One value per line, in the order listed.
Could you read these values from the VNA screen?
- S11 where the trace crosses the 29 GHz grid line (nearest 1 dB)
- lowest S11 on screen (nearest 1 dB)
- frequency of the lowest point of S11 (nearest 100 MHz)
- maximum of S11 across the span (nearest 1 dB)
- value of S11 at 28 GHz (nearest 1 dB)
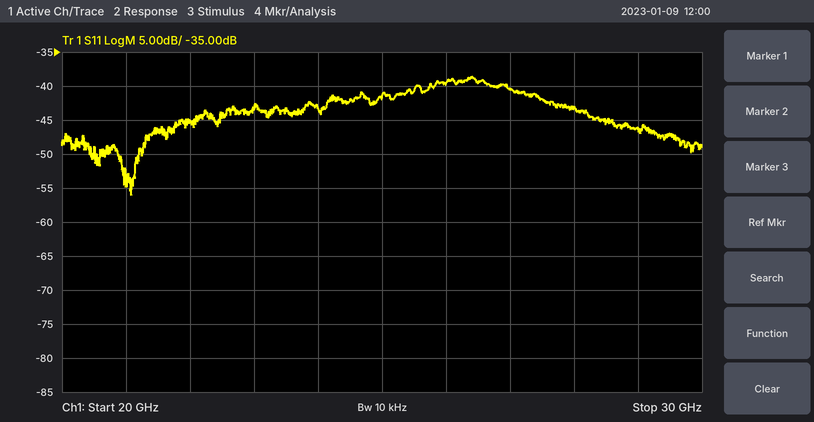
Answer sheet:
-46 dB
-56 dB
21.1 GHz
-39 dB
-43 dB
